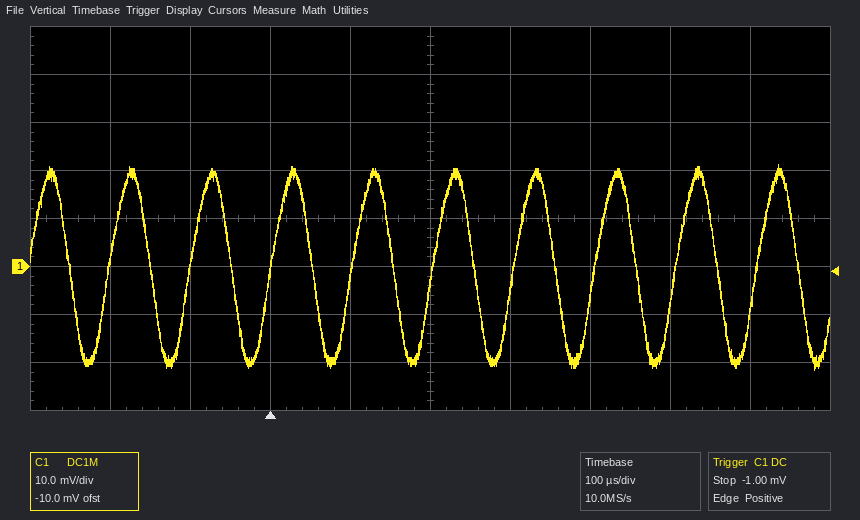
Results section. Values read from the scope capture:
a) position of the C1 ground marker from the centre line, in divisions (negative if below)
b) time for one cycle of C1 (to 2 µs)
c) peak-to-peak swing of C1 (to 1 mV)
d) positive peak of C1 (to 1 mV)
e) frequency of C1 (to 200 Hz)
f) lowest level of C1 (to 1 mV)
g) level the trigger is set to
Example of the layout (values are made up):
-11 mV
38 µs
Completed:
-1.0 div
102 µs
43 mV
21 mV
9.8 kHz
-22 mV
-1.00 mV
